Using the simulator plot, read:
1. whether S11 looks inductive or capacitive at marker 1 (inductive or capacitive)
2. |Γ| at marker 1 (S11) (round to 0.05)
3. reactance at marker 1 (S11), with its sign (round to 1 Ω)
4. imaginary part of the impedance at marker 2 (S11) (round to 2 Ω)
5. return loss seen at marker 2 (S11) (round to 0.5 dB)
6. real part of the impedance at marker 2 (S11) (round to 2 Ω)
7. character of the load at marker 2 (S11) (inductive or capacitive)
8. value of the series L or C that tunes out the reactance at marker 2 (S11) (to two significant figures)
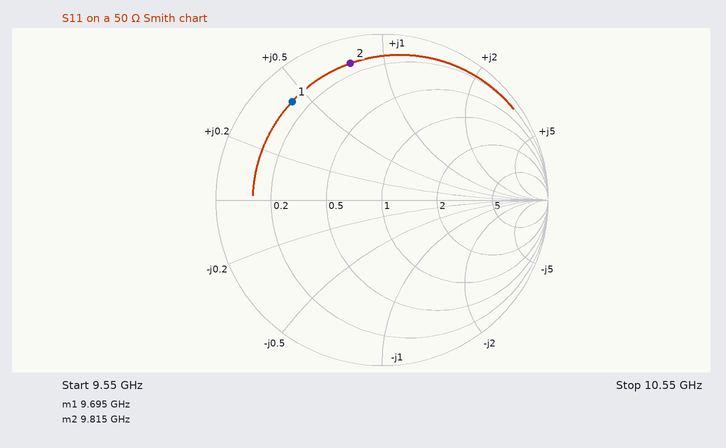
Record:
inductive
0.80
+22 Ω
+40 Ω
1.5 dB
6 Ω
inductive
410 fF
